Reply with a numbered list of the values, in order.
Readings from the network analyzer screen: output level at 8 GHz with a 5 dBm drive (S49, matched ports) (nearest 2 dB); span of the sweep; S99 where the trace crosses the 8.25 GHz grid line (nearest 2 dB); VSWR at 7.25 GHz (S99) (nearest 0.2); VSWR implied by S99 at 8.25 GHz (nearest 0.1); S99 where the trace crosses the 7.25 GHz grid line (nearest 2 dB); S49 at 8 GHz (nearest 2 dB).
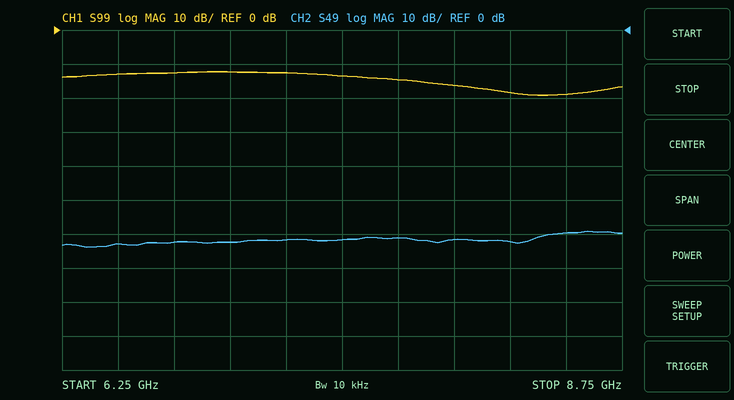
1. -56 dBm
2. 2.5 GHz
3. -18 dB
4. 1.6
5. 1.3
6. -12 dB
7. -62 dB
